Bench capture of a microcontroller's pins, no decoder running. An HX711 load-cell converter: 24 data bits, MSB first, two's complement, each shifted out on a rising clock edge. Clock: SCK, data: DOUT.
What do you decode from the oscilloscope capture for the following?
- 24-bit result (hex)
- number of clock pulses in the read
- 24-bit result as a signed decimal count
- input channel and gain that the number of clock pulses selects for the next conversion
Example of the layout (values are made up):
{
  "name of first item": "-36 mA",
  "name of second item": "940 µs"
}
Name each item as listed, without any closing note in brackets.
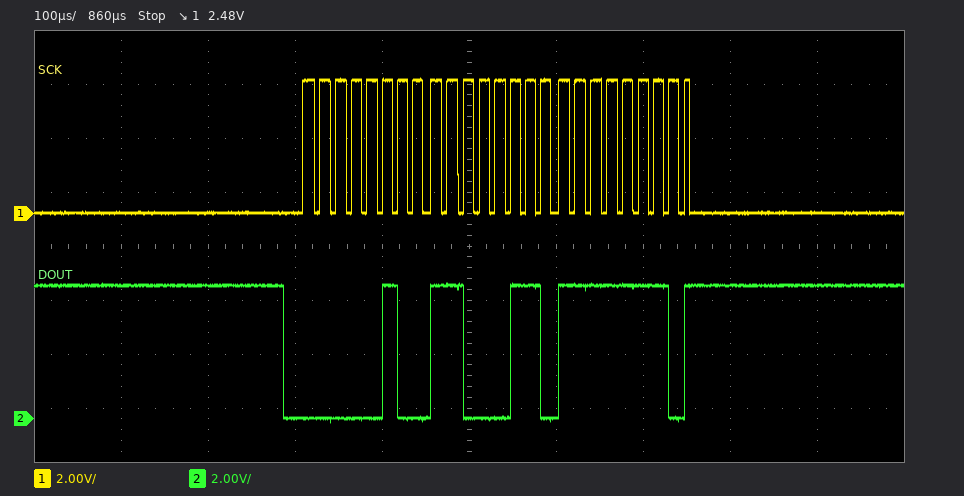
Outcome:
{
  "24-bit result": "0x04C6FE",
  "number of clock pulses in the read": "25",
  "24-bit result as a signed decimal count": "313086",
  "input channel and gain that the number of clock pulses selects for the next conversion": "channel A, gain 128"
}
